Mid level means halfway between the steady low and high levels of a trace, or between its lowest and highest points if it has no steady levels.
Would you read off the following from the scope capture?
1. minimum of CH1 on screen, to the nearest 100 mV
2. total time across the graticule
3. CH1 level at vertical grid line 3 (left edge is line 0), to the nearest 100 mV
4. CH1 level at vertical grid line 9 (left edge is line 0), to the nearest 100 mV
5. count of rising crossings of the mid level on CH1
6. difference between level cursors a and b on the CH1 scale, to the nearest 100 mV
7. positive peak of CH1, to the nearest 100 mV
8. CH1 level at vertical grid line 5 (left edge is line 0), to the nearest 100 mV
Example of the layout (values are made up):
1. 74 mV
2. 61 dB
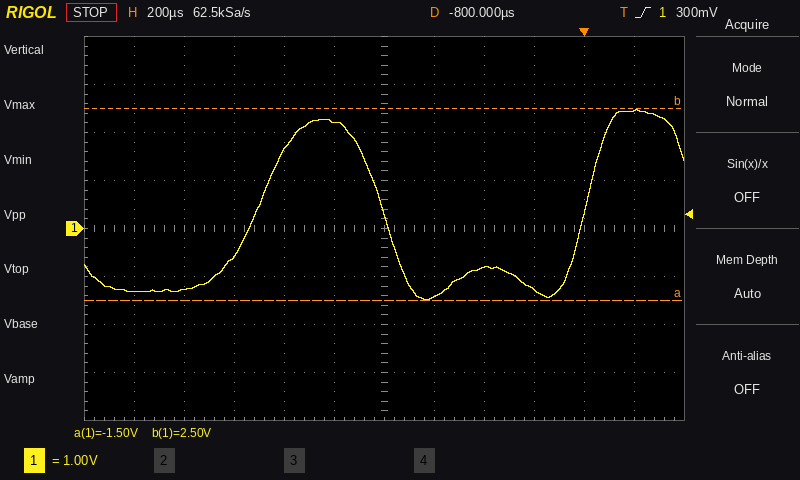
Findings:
1. -1.5 V
2. 2.4 ms
3. -600 mV
4. -1.3 V
5. 2
6. 4.0 V
7. 2.5 V
8. 2.2 V
